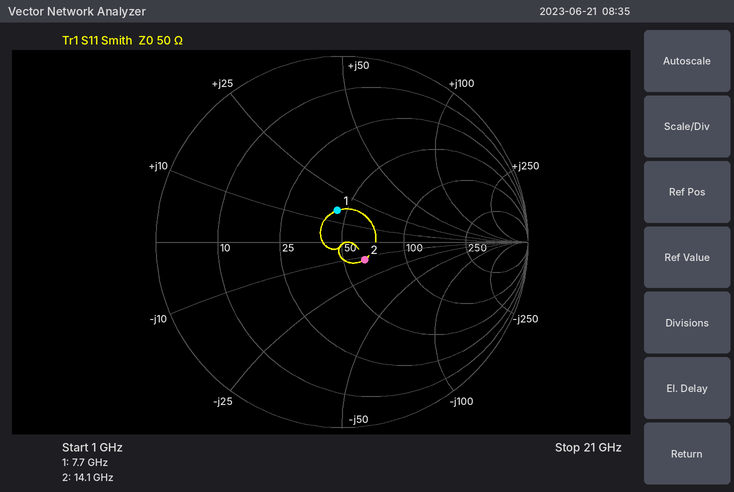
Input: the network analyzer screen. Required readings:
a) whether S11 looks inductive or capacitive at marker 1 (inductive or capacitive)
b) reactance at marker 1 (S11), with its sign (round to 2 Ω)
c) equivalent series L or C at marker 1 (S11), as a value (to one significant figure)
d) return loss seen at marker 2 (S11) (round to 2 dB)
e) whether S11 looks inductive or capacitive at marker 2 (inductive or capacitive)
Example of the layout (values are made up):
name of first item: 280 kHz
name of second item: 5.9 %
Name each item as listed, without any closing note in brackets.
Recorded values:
whether S11 looks inductive or capacitive at marker 1: inductive
reactance at marker 1 (S11), with its sign: +16 Ω
equivalent series L or C at marker 1 (S11), as a value: 300 pH
return loss seen at marker 2 (S11): 16 dB
whether S11 looks inductive or capacitive at marker 2: capacitive
